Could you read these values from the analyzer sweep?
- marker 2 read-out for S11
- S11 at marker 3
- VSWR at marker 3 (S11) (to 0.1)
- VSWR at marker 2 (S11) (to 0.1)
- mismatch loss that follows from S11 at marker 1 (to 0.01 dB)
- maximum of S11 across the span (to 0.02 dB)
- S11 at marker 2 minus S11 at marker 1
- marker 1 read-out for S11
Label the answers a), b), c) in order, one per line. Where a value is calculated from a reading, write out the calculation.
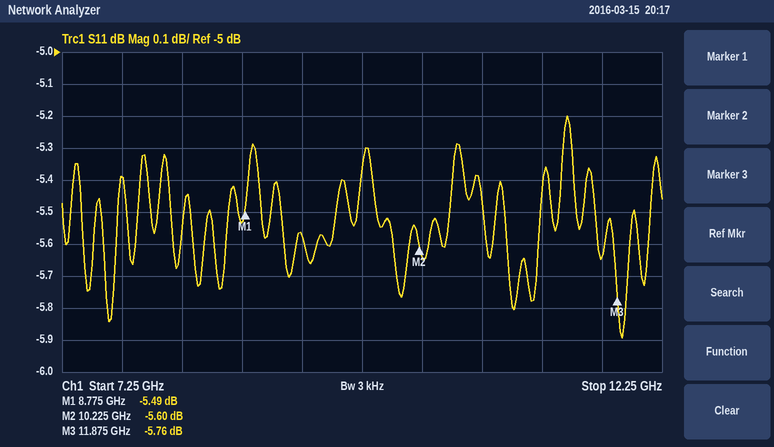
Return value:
a) -5.60 dB
b) -5.76 dB
c) (1 + 0.5152)/(1 − 0.5152) ≈ 3.1
d) (1 + 0.5248)/(1 − 0.5248) ≈ 3.2
e) −10 log10(1 − 10^(-5.49/10)) ≈ 1.44 dB
f) -5.20 dB
g) -5.6 − (-5.49) = -0.11 dB
h) -5.49 dB
